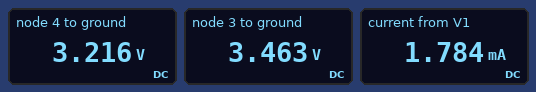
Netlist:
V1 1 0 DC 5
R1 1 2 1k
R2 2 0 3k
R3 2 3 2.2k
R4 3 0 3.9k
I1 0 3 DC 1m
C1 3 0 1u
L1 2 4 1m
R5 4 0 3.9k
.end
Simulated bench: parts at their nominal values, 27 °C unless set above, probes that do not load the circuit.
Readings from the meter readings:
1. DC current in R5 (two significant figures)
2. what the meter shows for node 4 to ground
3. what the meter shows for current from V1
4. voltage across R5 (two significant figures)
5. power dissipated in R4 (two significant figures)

820 µA
3.216 V
1.784 mA
3.2 V
3.1 mW
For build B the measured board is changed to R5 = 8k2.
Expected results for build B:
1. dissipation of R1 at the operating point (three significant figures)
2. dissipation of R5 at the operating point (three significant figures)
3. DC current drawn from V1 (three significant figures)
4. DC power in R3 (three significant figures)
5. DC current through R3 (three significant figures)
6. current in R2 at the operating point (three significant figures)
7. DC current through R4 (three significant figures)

2.30 mW
1.48 mW
1.52 mA
10.3 µW
68.4 µA
1.16 mA
932 µA
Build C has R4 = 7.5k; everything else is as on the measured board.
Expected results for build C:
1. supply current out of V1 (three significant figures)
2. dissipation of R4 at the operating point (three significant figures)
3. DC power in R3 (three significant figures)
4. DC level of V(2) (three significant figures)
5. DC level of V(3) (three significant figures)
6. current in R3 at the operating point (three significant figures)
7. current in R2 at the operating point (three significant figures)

1.59 mA
2.51 mW
391 µW
3.41 V
4.34 V
422 µA
1.14 mA
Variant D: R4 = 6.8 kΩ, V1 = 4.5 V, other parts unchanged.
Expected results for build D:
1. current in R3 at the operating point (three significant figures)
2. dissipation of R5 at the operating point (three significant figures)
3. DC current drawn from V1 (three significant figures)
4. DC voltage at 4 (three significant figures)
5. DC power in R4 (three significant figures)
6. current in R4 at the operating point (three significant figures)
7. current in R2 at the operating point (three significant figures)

412 µA
2.45 mW
1.41 mA
3.09 V
2.35 mW
588 µA
1.03 mA
